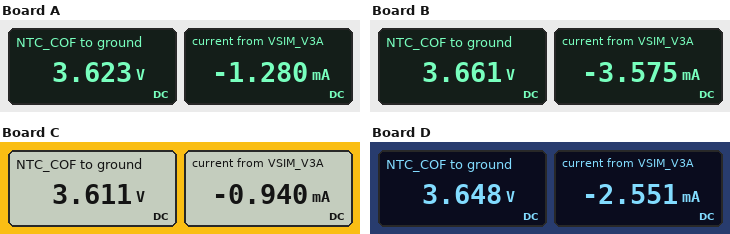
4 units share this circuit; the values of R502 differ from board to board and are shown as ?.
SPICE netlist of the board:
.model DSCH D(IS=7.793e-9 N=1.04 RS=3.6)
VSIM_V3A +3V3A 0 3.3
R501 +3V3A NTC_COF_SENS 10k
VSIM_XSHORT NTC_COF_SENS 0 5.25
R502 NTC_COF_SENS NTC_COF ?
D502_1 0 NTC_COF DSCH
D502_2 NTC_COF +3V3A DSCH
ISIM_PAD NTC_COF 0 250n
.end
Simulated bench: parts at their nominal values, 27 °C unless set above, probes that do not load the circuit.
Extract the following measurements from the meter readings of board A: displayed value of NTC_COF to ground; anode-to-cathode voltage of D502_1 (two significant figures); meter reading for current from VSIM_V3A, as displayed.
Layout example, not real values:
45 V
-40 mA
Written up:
3.623 V
-3.6 V
-1.280 mA
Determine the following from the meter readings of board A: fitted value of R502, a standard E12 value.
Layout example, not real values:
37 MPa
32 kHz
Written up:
1.5 kΩ
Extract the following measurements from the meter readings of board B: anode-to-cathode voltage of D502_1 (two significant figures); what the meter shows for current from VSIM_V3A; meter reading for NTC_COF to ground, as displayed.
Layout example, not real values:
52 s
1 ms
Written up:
-3.7 V
-3.575 mA
3.661 V
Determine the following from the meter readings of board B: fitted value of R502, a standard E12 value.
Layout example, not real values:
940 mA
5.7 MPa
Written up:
470 Ω
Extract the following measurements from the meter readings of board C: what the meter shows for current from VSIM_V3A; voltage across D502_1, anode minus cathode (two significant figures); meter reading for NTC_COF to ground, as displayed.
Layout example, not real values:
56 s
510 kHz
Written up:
-0.940 mA
-3.6 V
3.611 V
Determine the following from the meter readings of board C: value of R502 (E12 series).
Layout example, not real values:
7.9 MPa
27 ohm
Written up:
2.2 kΩ
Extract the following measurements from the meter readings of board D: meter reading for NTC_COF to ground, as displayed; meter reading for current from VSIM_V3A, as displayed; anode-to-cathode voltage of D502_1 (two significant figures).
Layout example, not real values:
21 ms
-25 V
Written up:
3.648 V
-2.551 mA
-3.6 V
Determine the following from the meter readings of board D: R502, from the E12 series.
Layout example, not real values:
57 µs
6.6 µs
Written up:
680 Ω
